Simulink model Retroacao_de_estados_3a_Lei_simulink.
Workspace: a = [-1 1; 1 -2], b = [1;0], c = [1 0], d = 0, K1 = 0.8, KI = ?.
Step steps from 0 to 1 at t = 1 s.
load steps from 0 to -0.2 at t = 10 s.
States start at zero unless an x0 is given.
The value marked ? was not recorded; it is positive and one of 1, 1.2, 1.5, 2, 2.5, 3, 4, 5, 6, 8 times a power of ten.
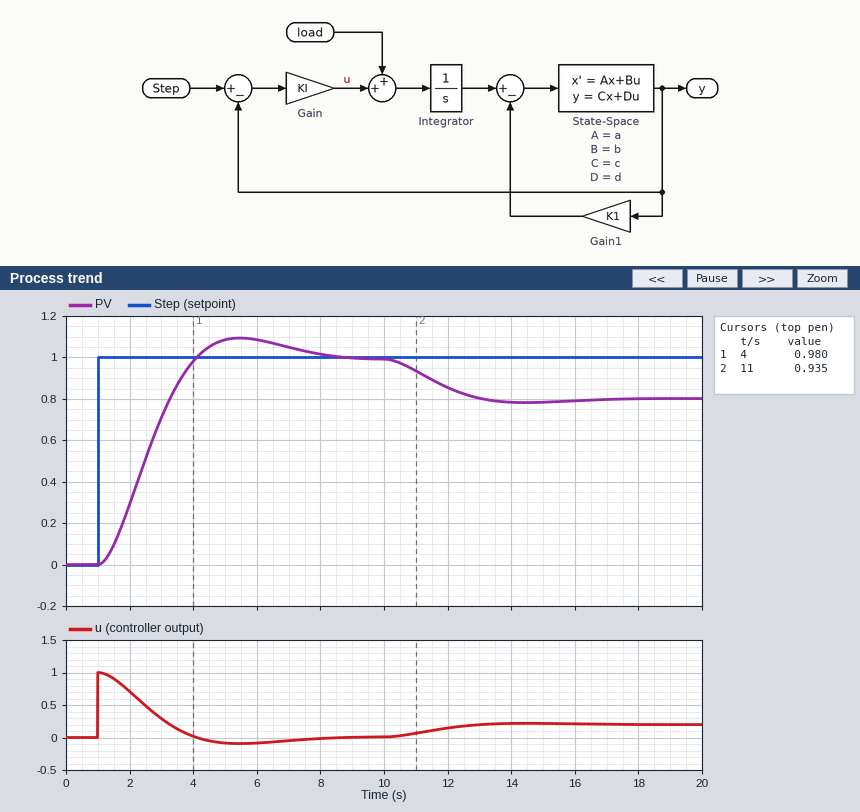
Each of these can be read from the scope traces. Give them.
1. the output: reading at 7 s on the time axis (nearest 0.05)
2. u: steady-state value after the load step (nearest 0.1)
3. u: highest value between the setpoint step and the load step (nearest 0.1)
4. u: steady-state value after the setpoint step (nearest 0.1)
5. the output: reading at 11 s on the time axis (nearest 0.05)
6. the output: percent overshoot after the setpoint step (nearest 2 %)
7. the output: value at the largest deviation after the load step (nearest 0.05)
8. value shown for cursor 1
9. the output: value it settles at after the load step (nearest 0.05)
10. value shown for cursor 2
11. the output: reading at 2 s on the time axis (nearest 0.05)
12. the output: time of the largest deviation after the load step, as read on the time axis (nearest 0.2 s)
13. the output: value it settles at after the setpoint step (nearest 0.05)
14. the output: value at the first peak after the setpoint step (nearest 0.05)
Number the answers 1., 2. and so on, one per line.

1. 1.05
2. 0.2
3. 1.0
4. 0.0
5. 0.95
6. 10 %
7. 0.80
8. 0.980
9. 0.80
10. 0.935
11. 0.30
12. 14.4 s
13. 1.00
14. 1.10
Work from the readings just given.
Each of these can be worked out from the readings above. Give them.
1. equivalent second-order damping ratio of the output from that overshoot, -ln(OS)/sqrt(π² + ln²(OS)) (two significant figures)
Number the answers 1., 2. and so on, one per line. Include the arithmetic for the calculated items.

1. ln(0.1) = -2.303; 2.303 / sqrt(9.870 + 5.302) = 0.59
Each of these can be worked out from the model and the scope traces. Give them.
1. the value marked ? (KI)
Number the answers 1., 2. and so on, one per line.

1. 1
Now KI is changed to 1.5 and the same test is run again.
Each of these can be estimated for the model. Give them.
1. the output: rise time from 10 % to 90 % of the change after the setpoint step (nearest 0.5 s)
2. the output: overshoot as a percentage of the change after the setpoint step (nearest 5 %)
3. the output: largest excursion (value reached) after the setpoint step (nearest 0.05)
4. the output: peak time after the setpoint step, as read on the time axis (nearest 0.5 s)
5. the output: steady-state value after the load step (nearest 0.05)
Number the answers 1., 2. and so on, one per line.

1. 1.5 s
2. 15 %
3. 1.15
4. 4.5 s
5. 0.85
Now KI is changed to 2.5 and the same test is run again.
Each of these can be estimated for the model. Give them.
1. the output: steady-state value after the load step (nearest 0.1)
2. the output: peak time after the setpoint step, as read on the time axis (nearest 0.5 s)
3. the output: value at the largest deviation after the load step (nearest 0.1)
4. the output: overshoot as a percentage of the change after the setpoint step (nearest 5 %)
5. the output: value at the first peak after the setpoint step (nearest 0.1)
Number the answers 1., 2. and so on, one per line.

1. 0.9
2. 3.5 s
3. 0.9
4. 25 %
5. 1.2
